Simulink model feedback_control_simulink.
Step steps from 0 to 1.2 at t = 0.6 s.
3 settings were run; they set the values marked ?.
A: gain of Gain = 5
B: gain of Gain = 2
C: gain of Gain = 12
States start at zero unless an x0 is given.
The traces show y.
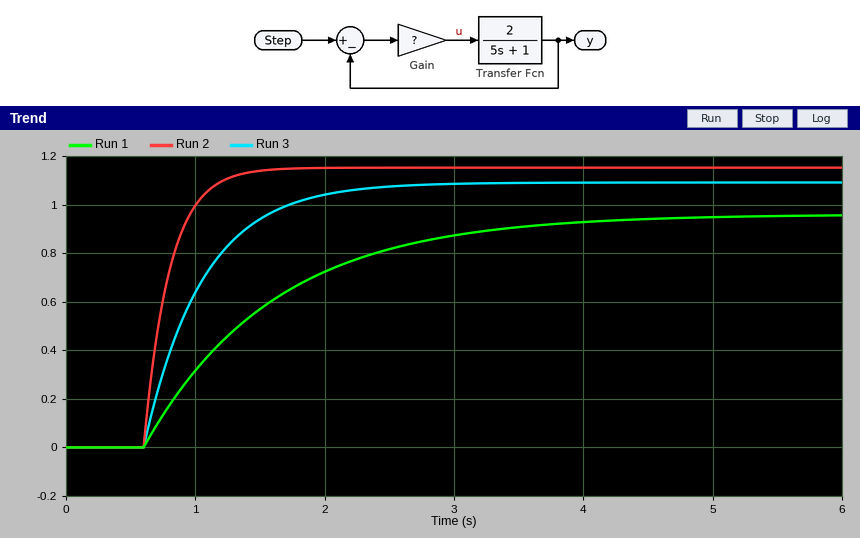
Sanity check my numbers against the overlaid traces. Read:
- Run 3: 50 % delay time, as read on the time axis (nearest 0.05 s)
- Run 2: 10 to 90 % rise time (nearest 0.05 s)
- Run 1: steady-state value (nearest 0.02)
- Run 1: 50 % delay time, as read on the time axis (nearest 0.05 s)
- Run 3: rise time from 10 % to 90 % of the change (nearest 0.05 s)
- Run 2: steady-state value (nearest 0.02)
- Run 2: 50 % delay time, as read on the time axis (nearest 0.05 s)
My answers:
0.90 s
0.45 s
0.96
1.30 s
1.00 s
1.16
0.75 s
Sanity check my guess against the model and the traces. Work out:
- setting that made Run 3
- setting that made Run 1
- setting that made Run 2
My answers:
A
B
C
